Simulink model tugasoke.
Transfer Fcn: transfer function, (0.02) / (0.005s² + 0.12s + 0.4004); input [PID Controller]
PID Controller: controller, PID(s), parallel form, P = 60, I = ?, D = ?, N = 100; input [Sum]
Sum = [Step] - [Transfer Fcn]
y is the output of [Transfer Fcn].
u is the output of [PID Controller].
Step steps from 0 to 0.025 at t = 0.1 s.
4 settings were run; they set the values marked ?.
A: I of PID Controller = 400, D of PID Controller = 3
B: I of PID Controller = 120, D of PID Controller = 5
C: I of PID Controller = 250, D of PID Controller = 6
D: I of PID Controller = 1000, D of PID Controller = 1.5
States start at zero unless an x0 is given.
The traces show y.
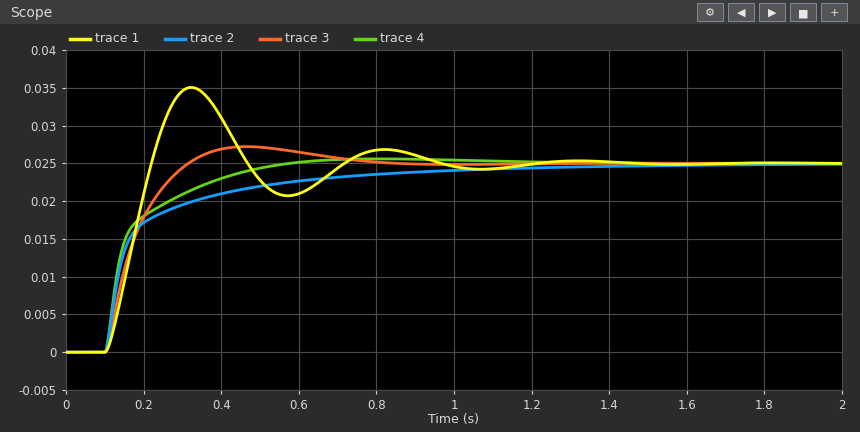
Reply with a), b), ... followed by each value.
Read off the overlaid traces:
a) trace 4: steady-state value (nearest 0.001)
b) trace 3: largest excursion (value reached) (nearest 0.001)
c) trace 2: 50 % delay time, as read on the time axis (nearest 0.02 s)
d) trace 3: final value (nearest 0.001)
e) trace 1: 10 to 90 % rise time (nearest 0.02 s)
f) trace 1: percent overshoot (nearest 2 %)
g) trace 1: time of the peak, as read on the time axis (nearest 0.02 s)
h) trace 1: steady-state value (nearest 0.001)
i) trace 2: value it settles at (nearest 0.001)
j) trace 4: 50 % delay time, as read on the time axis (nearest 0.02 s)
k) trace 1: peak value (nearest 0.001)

a) 0.025
b) 0.027
c) 0.14 s
d) 0.025
e) 0.08 s
f) 40 %
g) 0.32 s
h) 0.025
i) 0.025
j) 0.14 s
k) 0.035
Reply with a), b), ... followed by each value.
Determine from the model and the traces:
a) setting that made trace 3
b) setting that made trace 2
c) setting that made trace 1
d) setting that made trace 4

a) A
b) B
c) D
d) C
